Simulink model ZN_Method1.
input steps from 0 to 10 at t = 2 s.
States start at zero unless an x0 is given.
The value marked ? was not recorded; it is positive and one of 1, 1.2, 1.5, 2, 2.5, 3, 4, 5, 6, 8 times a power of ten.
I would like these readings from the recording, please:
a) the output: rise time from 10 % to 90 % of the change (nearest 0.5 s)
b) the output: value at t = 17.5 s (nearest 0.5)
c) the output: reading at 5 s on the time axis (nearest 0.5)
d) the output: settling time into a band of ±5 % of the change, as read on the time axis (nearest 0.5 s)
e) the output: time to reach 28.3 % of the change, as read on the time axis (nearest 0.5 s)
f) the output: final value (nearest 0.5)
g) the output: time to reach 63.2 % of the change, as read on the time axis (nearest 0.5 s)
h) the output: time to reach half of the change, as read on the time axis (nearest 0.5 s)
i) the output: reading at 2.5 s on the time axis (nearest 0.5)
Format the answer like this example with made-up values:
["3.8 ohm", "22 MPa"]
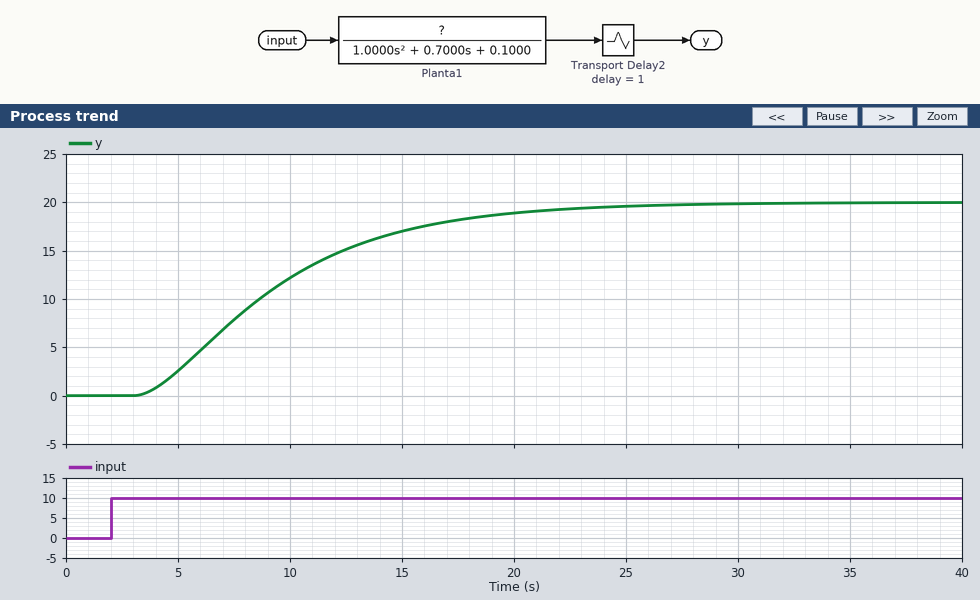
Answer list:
["12.5 s", "18.0", "2.5", "20.5 s", "6.5 s", "20.0", "10.5 s", "8.5 s", "0.0"]
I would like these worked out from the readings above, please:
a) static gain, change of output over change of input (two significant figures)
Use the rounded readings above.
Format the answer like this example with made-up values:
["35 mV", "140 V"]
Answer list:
["2.0"]
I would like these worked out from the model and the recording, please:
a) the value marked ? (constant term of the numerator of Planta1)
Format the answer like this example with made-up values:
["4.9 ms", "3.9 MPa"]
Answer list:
["0.2"]
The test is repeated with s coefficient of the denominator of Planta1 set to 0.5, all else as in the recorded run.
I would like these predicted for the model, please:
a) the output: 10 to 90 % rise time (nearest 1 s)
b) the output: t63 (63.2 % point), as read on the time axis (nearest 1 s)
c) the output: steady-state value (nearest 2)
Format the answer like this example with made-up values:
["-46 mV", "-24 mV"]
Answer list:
["8 s", "9 s", "20"]
